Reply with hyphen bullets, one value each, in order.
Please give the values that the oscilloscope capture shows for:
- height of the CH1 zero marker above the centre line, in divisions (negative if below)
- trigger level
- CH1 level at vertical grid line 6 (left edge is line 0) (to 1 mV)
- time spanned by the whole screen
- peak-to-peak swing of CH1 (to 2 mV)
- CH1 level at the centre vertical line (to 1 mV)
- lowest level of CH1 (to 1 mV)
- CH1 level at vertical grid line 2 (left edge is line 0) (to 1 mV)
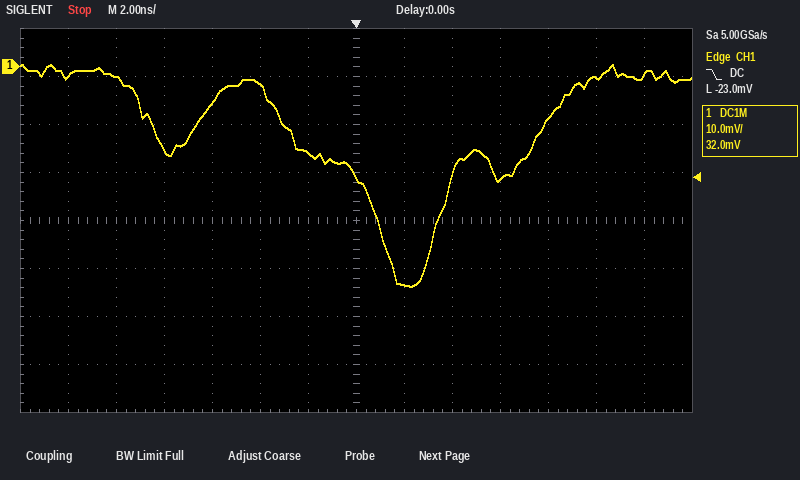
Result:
- +3.2 div
- -23.0 mV
- -18 mV
- 28 ns
- 46 mV
- -23 mV
- -46 mV
- -2 mV
